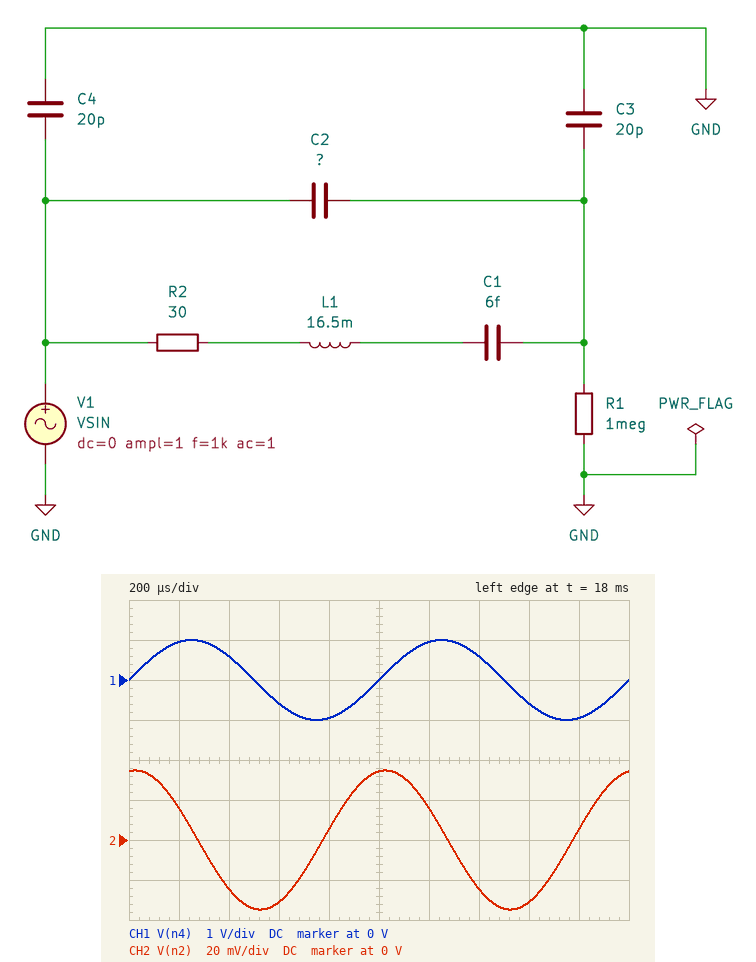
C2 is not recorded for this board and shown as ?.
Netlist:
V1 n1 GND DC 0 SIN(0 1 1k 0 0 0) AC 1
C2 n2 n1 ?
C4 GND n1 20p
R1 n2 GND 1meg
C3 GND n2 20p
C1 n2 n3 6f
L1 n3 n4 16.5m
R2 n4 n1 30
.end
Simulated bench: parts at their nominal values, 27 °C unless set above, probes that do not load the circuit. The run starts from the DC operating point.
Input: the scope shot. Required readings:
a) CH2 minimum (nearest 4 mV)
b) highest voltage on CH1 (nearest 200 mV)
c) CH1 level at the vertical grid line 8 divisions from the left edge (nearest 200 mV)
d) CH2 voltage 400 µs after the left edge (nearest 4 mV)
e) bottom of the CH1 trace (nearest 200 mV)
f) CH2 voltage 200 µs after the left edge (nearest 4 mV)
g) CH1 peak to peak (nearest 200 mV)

-36 mV
1.0 V
-600 mV
-24 mV
-1.0 V
16 mV
2.0 V
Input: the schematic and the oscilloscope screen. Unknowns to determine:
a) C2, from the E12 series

5.6 pF
